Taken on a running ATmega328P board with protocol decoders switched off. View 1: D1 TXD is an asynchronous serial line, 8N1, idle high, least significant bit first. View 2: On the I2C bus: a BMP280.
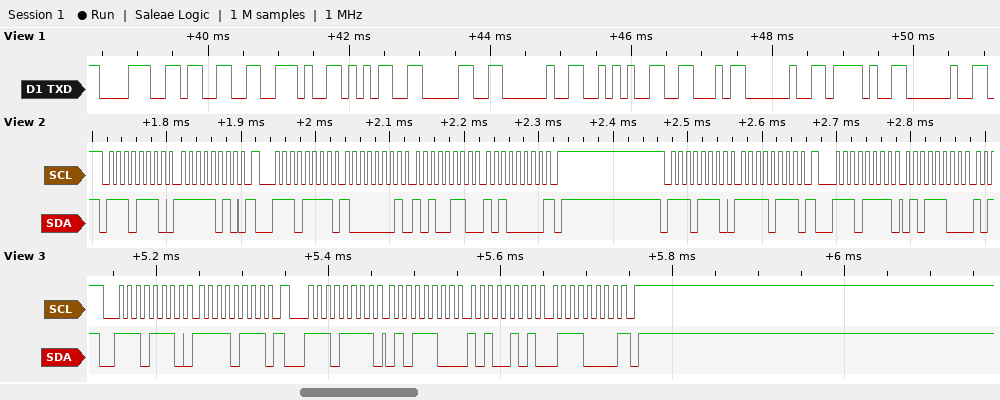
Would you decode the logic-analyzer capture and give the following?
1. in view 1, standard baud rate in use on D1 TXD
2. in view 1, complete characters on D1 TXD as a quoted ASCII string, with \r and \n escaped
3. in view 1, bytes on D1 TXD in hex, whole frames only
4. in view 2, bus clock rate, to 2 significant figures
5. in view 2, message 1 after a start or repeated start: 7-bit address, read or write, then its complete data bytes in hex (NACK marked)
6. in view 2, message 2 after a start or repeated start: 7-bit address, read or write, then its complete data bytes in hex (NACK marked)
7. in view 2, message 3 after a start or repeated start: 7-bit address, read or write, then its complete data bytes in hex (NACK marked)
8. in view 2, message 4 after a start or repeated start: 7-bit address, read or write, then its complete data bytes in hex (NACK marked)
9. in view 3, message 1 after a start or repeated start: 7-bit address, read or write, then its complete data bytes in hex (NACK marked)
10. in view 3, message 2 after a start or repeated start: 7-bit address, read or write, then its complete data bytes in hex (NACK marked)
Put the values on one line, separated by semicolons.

9600 baud; "83.50 *F / "; 38 33 2E 35 30 20 2A 46 20 2F 20; 100 kHz; 0x77 write: FA; 0x77 read: 81 A6 A0 NACK; 0x77 write: F7; 0x77 read: 5C; 0x77 write: F7; 0x77 read: 5C A5 70 NACK
